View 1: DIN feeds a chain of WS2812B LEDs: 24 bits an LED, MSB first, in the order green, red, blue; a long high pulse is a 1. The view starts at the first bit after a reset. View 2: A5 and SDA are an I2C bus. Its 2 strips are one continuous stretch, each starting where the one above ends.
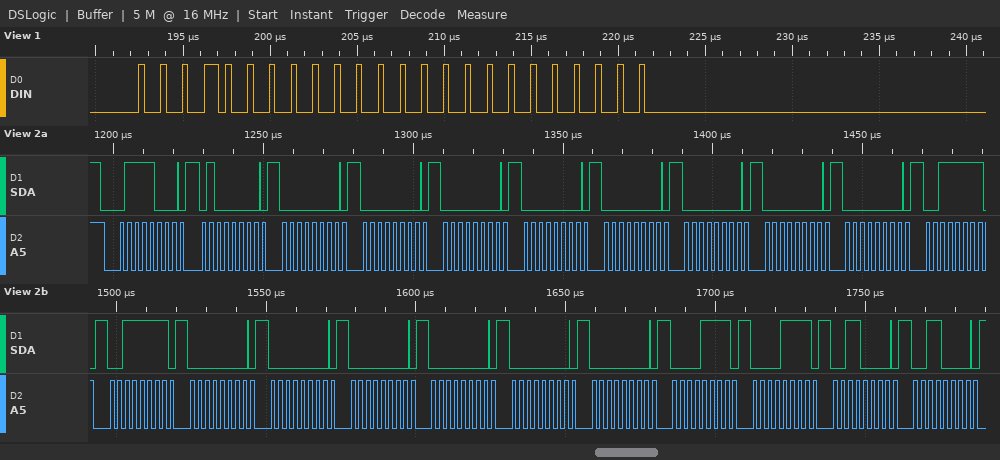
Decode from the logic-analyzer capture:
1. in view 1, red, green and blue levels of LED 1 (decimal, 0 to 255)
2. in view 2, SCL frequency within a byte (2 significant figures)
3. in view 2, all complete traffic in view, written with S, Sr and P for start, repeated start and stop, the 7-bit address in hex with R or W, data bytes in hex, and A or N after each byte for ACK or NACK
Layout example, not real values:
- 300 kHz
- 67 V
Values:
- 0, 16, 0
- 400 kHz
- S 3CW A 40 A 00 A 00 A 00 A 00 A 00 A 00 A 00 A 00 A 3F A 3F A 00 A 00 A 00 A 00 A 00 A 00 A 0F A 0F A 30 A 30 A
